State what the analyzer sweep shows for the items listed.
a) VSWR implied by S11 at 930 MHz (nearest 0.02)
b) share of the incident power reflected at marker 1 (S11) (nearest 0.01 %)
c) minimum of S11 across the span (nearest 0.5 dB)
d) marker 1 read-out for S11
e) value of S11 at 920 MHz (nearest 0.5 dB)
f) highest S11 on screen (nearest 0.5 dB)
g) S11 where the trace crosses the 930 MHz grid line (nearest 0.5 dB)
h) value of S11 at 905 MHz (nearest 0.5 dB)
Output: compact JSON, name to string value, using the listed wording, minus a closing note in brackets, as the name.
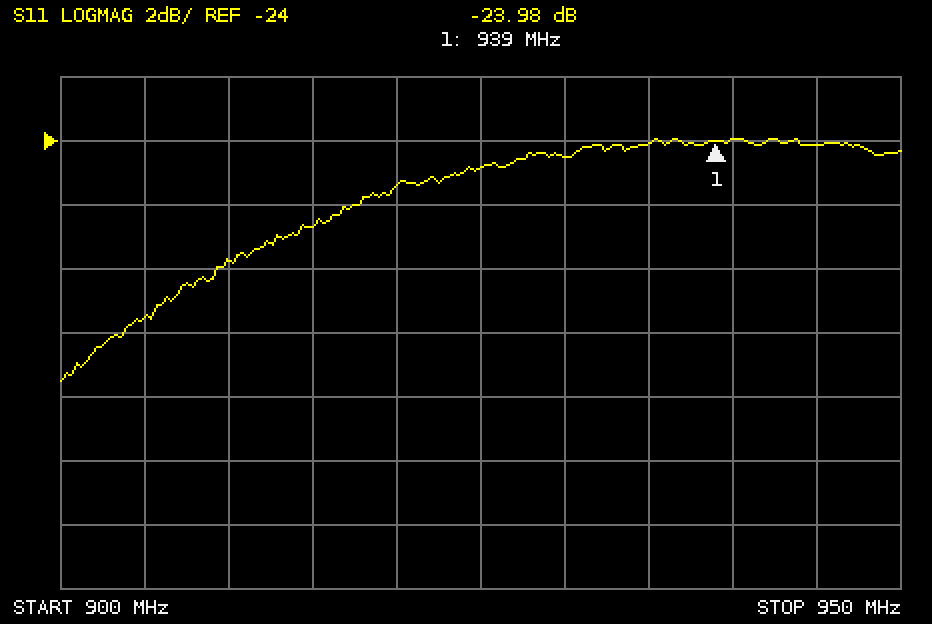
{"VSWR implied by S11 at 930 MHz": "1.12", "share of the incident power reflected at marker 1 (S11)": "0.40 %", "minimum of S11 across the span": "-31.5 dB", "marker 1 read-out for S11": "-23.98 dB", "value of S11 at 920 MHz": "-25.5 dB", "highest S11 on screen": "-24.0 dB", "S11 where the trace crosses the 930 MHz grid line": "-24.5 dB", "value of S11 at 905 MHz": "-29.5 dB"}
